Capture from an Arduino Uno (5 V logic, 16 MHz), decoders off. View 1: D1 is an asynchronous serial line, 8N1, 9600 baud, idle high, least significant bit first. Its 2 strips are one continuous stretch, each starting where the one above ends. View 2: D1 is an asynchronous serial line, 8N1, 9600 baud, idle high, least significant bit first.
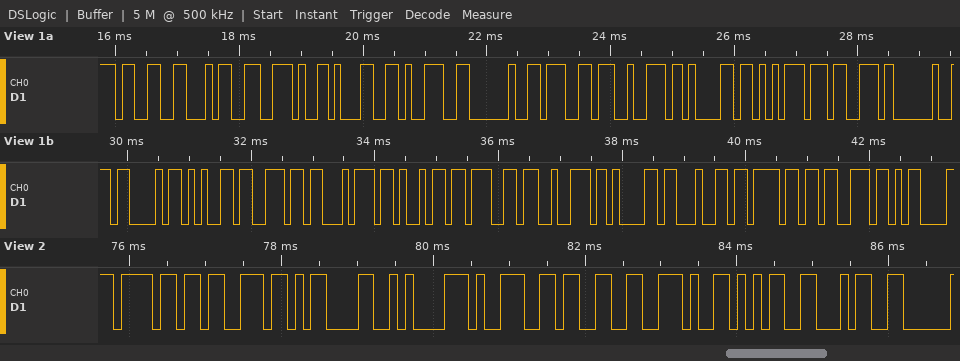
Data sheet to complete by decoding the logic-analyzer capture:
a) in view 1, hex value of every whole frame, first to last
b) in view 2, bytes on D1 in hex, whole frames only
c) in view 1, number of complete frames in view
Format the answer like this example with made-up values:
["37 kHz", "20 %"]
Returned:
["33 34 2E 31 39 20 67 72 61 75 73 20 43 65 6E 74 69 67 72 61 64 6F 73 0D", "6F 73 0D 0A 39 33 2E 35 34", "24"]
